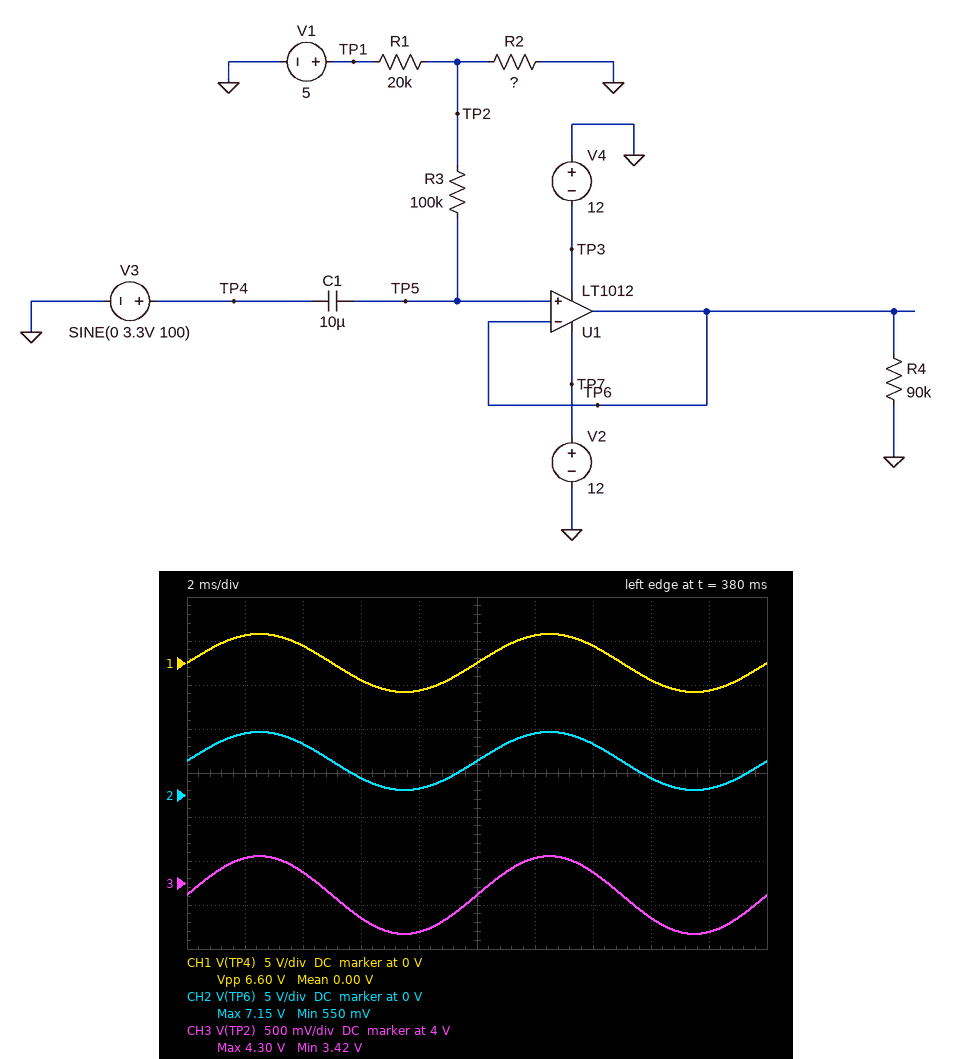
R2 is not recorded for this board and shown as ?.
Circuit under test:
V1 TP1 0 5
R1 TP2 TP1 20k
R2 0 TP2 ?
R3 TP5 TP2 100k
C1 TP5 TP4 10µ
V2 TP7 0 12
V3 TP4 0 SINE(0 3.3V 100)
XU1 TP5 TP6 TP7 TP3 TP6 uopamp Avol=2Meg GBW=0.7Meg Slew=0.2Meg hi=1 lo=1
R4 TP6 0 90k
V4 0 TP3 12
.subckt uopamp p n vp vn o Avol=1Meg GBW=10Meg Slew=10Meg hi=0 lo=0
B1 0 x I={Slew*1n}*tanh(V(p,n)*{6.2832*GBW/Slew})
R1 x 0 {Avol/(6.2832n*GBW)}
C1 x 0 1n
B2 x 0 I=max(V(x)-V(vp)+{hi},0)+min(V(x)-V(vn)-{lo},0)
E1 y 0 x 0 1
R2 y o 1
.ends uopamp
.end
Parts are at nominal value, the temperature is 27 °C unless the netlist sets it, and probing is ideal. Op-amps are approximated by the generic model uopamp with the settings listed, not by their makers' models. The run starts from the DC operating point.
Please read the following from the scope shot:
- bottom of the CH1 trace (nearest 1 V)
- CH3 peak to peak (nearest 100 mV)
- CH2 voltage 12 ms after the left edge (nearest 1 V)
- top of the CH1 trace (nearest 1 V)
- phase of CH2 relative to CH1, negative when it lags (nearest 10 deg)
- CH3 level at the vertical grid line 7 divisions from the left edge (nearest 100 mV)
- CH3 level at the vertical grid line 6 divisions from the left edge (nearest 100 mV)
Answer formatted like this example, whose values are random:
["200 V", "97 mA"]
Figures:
["-3 V", "900 mV", "7 V", "3 V", "0 deg", "4.1 V", "4.3 V"]
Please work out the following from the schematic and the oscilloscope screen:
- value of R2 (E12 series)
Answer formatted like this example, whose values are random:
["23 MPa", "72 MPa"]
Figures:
["68 kΩ"]
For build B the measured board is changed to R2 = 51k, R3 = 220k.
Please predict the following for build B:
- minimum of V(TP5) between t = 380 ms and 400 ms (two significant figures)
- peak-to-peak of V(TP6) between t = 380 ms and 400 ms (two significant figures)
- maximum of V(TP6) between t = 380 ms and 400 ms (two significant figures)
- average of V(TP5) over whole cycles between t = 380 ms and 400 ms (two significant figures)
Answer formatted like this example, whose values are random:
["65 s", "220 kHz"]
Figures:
["290 mV", "6.6 V", "6.9 V", "3.6 V"]
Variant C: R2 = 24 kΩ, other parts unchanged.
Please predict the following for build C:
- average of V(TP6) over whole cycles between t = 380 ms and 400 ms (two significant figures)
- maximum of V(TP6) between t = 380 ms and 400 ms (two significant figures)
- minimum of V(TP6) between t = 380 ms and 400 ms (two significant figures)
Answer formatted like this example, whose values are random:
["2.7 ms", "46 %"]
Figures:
["2.7 V", "6.0 V", "-580 mV"]
